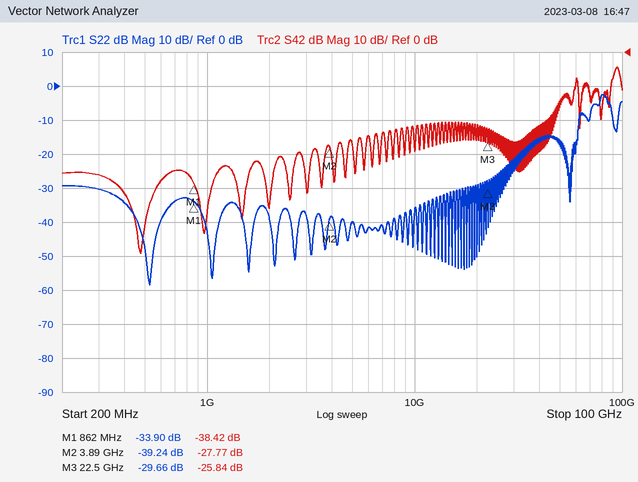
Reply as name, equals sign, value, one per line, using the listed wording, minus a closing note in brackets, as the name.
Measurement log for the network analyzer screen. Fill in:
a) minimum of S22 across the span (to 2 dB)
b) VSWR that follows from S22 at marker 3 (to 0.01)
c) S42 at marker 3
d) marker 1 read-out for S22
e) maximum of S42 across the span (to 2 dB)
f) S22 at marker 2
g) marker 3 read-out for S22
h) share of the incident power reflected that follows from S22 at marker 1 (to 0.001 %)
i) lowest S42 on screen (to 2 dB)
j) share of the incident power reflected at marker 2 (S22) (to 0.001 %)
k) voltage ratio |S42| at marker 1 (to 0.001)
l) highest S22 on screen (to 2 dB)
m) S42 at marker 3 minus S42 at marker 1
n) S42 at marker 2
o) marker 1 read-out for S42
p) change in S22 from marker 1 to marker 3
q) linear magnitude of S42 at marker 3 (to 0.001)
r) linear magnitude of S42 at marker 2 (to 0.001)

minimum of S22 across the span = -58 dB
VSWR that follows from S22 at marker 3 = 1.07
S42 at marker 3 = -25.84 dB
marker 1 read-out for S22 = -33.90 dB
maximum of S42 across the span = -4 dB
S22 at marker 2 = -39.24 dB
marker 3 read-out for S22 = -29.66 dB
share of the incident power reflected that follows from S22 at marker 1 = 0.041 %
lowest S42 on screen = -60 dB
share of the incident power reflected at marker 2 (S22) = 0.012 %
voltage ratio |S42| at marker 1 = 0.012
highest S22 on screen = -2 dB
S42 at marker 3 minus S42 at marker 1 = 12.58 dB
S42 at marker 2 = -27.77 dB
marker 1 read-out for S42 = -38.42 dB
change in S22 from marker 1 to marker 3 = 4.24 dB
linear magnitude of S42 at marker 3 = 0.051
linear magnitude of S42 at marker 2 = 0.041
